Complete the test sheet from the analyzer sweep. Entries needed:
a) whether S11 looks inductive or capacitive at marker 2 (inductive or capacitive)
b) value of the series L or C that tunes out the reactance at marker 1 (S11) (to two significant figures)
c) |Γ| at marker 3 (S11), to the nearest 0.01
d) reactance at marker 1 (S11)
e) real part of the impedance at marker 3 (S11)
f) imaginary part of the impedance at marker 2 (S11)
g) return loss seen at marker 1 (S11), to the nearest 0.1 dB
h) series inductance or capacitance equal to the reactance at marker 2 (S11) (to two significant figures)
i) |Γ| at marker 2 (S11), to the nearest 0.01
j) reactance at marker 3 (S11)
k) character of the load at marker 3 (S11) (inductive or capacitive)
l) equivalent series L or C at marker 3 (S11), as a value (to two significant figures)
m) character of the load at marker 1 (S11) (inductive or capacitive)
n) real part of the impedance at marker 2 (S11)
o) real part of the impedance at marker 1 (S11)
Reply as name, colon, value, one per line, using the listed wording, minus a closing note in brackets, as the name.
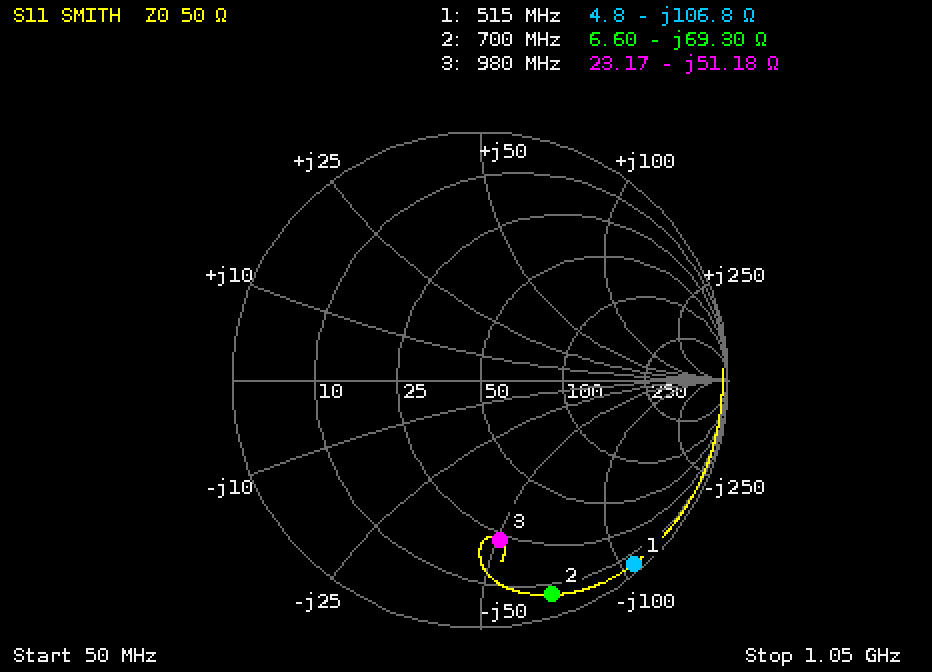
whether S11 looks inductive or capacitive at marker 2: capacitive
value of the series L or C that tunes out the reactance at marker 1 (S11): 33 nH
|Γ| at marker 3 (S11), to the nearest 0.01: 0.65
reactance at marker 1: -106.8 Ω
real part of the impedance at marker 3: 23.17 Ω
imaginary part of the impedance at marker 2: -69.30 Ω
return loss seen at marker 1 (S11), to the nearest 0.1 dB: 0.3 dB
series inductance or capacitance equal to the reactance at marker 2 (S11): 3.3 pF
|Γ| at marker 2 (S11), to the nearest 0.01: 0.91
reactance at marker 3: -51.18 Ω
character of the load at marker 3 (S11): capacitive
equivalent series L or C at marker 3 (S11), as a value: 3.2 pF
character of the load at marker 1 (S11): capacitive
real part of the impedance at marker 2: 6.60 Ω
real part of the impedance at marker 1: 4.8 Ω
